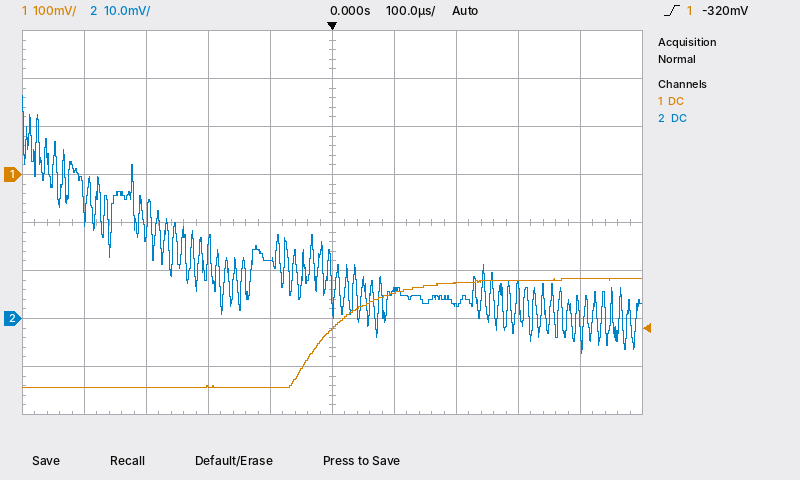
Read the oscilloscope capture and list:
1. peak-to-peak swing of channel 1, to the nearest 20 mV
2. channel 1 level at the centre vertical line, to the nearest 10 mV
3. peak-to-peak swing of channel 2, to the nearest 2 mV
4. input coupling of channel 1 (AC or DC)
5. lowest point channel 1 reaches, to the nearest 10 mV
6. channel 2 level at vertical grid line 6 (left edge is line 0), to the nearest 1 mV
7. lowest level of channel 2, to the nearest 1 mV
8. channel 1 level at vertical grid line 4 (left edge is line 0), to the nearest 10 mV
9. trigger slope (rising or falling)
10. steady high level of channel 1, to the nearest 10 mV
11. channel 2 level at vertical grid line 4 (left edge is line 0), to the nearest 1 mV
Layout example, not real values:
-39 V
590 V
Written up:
220 mV
-320 mV
54 mV
DC
-440 mV
6 mV
-7 mV
-440 mV
rising
-220 mV
12 mV
